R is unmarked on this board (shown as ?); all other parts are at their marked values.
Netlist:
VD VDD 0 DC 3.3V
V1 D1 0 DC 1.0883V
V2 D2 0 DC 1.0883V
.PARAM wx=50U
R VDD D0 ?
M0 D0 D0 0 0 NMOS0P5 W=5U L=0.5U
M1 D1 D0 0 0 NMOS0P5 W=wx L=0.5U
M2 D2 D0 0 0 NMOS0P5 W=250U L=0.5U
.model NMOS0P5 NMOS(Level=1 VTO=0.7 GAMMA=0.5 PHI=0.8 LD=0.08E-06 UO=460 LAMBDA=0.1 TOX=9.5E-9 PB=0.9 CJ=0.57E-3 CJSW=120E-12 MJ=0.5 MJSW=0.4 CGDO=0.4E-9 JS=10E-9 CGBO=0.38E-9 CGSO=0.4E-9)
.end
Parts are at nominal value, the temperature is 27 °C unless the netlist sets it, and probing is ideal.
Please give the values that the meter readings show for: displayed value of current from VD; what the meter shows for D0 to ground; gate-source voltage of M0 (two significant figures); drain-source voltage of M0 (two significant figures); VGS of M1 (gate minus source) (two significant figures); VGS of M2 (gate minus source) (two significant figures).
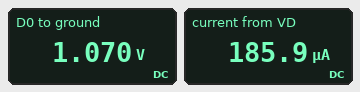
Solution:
185.9 µA
1.070 V
1.1 V
1.1 V
1.1 V
1.1 V
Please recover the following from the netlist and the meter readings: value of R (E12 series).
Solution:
12 kΩ
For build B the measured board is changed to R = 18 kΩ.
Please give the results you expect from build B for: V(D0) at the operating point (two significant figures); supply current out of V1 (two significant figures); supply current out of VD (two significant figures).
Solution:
1.0 V
1.3 mA
130 µA
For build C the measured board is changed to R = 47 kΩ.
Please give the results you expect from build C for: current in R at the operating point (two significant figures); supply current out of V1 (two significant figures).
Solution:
51 µA
520 µA
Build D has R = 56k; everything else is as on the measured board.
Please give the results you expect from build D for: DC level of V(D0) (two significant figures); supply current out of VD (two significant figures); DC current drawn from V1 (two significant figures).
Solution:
880 mV
43 µA
440 µA
